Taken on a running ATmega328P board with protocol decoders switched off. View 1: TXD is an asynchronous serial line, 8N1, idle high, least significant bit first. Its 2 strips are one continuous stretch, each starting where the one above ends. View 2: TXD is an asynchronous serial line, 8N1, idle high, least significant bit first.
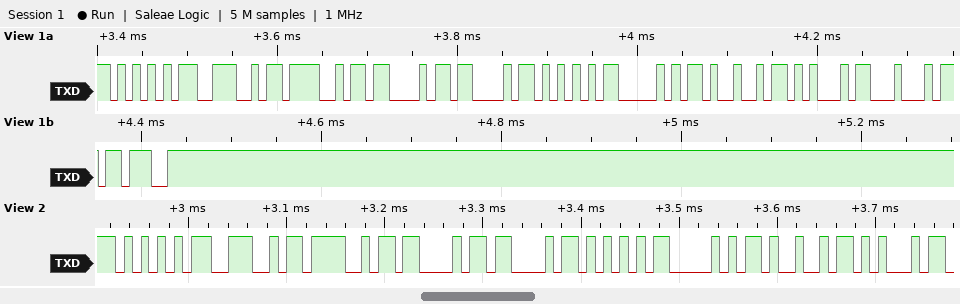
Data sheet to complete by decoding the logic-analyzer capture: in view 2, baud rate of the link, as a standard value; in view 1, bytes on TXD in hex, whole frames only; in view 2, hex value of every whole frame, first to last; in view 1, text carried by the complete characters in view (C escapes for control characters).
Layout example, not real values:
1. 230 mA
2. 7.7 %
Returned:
1. 115200 baud
2. 55 4E 4F 43 43 55 50 49 45 44 3B
3. 55 4E 4F 43 43 55 50 49 45
4. "UNOCCUPIED;"
